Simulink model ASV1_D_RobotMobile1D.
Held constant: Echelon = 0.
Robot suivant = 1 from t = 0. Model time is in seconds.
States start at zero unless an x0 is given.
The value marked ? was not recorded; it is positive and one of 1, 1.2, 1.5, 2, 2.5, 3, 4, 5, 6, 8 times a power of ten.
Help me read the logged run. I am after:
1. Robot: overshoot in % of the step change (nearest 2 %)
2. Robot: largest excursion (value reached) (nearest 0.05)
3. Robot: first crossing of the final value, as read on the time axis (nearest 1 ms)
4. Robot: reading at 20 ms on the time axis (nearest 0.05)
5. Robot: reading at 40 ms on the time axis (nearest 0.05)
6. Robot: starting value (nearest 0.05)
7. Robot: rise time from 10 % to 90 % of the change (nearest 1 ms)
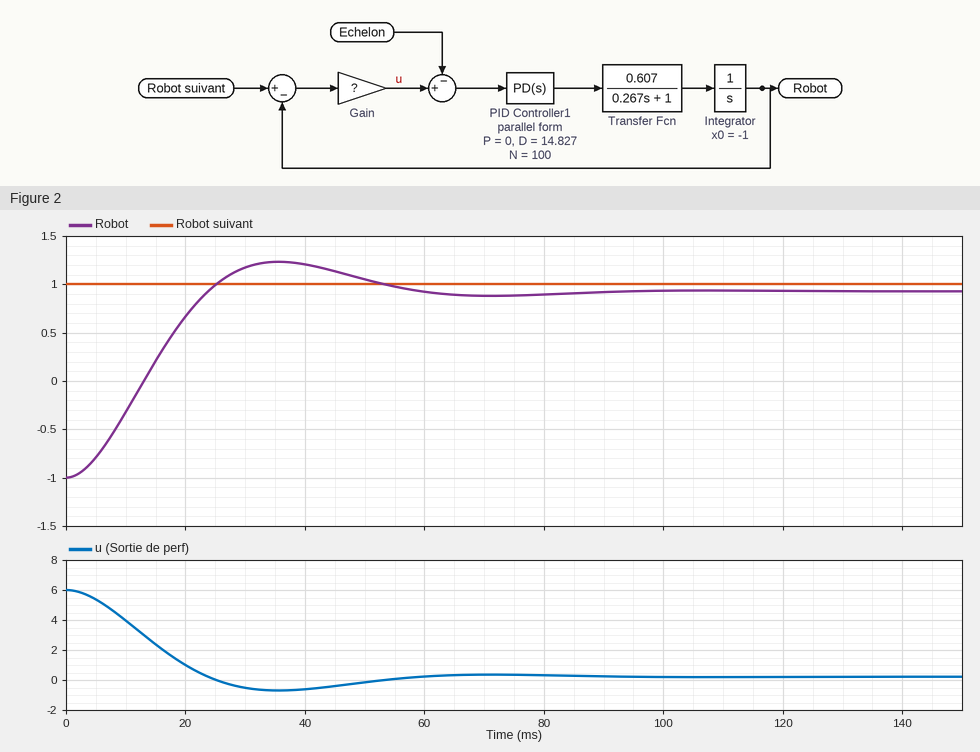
16 %
1.25
24 ms
0.65
1.20
-1.00
16 ms
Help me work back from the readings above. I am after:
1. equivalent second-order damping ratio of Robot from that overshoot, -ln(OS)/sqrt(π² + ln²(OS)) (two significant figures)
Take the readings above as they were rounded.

0.50
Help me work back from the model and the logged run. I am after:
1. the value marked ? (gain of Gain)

3
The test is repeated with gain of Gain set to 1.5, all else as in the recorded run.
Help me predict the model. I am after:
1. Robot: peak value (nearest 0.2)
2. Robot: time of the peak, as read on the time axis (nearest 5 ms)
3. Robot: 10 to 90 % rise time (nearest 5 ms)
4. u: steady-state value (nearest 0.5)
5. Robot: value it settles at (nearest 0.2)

1.0
60 ms
30 ms
0.0
0.8
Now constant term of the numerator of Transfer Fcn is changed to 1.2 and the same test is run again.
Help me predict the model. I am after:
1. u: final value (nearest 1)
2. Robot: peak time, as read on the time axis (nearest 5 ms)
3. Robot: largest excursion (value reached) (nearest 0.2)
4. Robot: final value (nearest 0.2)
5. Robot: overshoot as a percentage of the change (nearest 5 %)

0
25 ms
1.6
1.0
30 %
